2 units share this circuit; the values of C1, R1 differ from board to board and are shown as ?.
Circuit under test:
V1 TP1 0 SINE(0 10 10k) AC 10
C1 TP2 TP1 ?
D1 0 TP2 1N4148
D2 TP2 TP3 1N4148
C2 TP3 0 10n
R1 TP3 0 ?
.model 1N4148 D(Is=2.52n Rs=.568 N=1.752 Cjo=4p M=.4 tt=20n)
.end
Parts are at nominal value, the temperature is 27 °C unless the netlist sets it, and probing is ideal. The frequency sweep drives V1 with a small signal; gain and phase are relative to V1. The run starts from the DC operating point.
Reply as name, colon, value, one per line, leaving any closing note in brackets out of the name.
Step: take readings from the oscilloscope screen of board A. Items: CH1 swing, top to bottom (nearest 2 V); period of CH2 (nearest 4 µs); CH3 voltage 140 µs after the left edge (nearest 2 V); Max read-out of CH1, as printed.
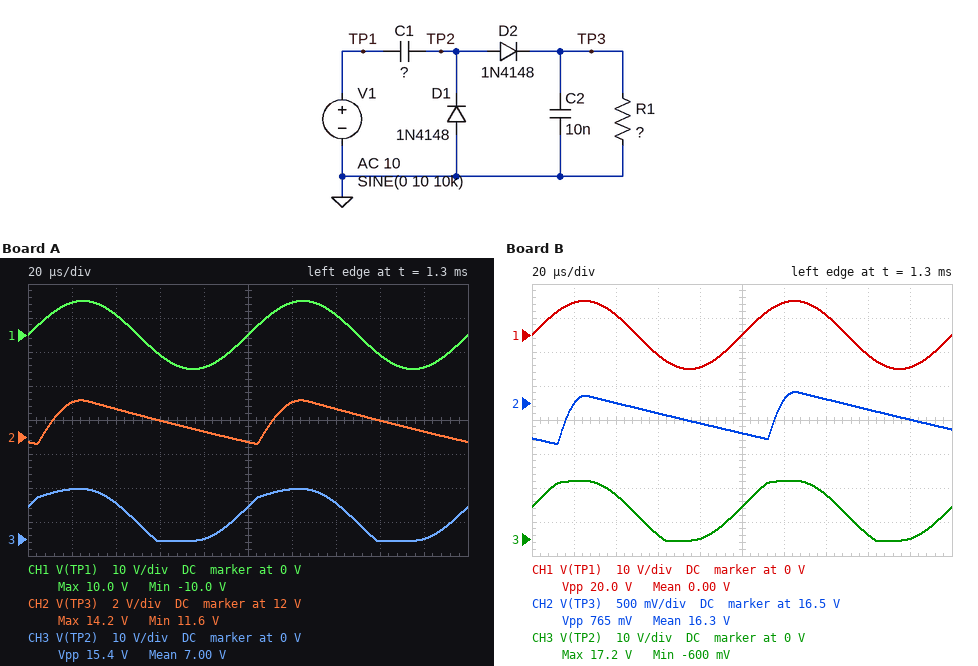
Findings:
CH1 swing, top to bottom: 20 V
period of CH2: 100 µs
CH3 voltage 140 µs after the left edge: 10 V
Max read-out of CH1, as printed: 10.0 V
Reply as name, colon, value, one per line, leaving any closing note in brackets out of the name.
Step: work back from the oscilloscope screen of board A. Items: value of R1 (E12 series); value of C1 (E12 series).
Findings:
value of R1: 39 kΩ
value of C1: 6.8 nF
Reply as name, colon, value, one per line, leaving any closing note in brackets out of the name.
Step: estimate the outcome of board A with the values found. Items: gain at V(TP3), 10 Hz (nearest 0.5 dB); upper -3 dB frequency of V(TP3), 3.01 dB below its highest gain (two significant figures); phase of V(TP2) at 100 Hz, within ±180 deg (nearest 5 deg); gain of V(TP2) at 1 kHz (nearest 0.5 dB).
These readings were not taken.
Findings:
gain at V(TP3), 10 Hz: -53.5 dB
upper -3 dB frequency of V(TP3), 3.01 dB below its highest gain: 430 Hz
phase of V(TP2) at 100 Hz, within ±180 deg: 0 deg
gain of V(TP2) at 1 kHz: 0 dB
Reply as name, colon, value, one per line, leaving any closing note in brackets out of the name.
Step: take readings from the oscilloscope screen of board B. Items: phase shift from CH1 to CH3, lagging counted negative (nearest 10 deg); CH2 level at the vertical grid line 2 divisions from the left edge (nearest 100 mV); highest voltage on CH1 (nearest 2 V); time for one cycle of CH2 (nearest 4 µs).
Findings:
phase shift from CH1 to CH3, lagging counted negative: 10 deg
CH2 level at the vertical grid line 2 divisions from the left edge: 16.5 V
highest voltage on CH1: 10 V
time for one cycle of CH2: 100 µs
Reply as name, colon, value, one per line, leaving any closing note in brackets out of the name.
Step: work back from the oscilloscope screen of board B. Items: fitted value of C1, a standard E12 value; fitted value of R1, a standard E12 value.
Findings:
fitted value of C1, a standard E12 value: 3.3 nF
fitted value of R1, a standard E12 value: 220 kΩ
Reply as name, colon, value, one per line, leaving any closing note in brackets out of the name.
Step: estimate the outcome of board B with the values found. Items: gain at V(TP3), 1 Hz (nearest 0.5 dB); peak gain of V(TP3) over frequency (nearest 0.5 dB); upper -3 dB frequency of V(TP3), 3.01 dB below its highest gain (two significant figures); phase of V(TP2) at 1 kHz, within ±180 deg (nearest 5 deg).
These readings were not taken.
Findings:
gain at V(TP3), 1 Hz: -53.0 dB
peak gain of V(TP3) over frequency: -39.0 dB
upper -3 dB frequency of V(TP3), 3.01 dB below its highest gain: 83 Hz
phase of V(TP2) at 1 kHz, within ±180 deg: 0 deg
